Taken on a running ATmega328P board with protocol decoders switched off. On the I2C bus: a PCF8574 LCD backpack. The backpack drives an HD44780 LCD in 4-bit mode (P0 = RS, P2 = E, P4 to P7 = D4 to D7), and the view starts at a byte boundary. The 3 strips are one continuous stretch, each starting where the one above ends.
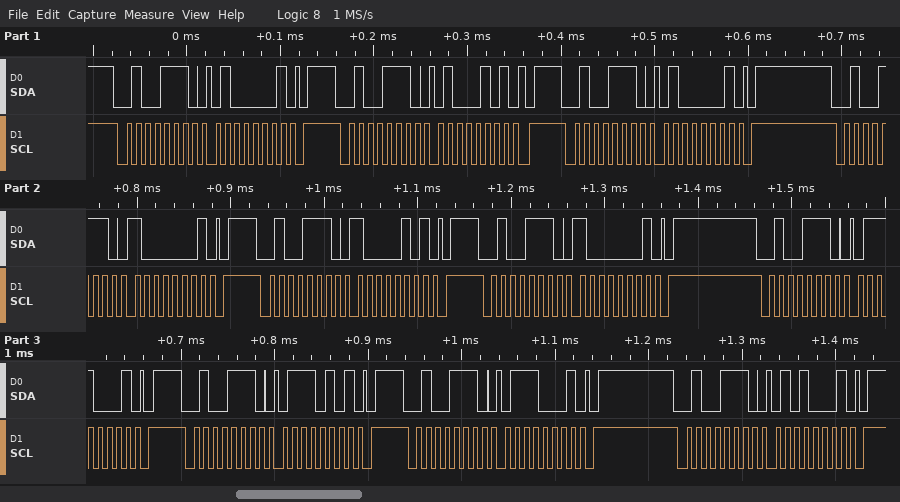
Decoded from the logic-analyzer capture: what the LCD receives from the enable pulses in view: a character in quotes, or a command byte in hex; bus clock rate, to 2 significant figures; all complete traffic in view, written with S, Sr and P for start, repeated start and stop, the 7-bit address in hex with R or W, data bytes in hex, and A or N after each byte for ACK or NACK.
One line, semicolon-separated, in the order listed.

'H'; 100 kHz; S 27W A 41 A P S 27W A 45 A P S 27W A 41 A P S 27W A 81 A P S 27W A 85 A P S 27W A 81 A P S 27W A 71 A P S 27W A 75 A P S 27W A 71 A P S 27W A 51 A P
